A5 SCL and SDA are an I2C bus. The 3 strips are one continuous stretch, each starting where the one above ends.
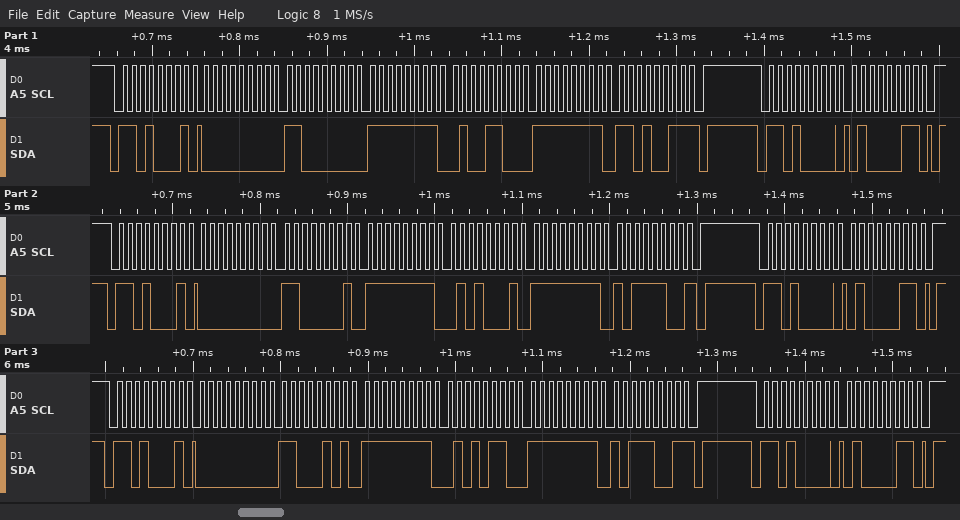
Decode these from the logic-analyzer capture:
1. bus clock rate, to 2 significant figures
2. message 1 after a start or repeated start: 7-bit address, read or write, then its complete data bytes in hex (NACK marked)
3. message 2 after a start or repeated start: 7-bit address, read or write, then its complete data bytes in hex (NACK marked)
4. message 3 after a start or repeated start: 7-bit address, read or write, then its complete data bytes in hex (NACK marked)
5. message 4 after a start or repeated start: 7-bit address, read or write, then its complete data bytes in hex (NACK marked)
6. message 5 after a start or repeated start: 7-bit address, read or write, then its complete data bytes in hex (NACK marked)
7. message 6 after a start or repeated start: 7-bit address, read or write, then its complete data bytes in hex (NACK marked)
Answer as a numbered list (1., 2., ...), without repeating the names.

1. 100 kHz
2. 0x68 read: 00 C0 FF 4C FF D3 NACK
3. 0x68 write: 43
4. 0x68 read: 00 C1 FF 51 FF BC NACK
5. 0x68 write: 43
6. 0x68 read: 00 C5 FF 56 FF B9 NACK
7. 0x68 write: 43
